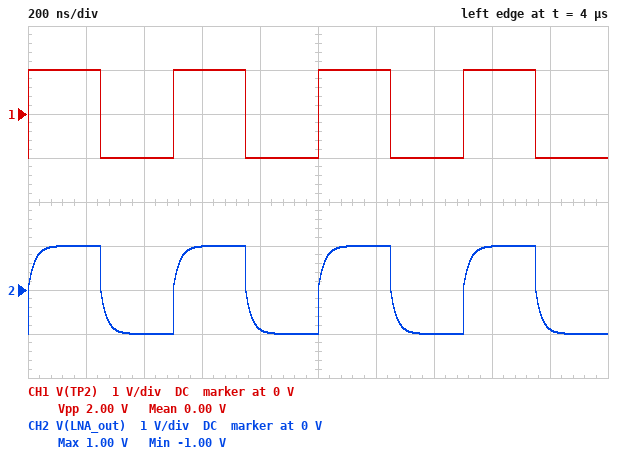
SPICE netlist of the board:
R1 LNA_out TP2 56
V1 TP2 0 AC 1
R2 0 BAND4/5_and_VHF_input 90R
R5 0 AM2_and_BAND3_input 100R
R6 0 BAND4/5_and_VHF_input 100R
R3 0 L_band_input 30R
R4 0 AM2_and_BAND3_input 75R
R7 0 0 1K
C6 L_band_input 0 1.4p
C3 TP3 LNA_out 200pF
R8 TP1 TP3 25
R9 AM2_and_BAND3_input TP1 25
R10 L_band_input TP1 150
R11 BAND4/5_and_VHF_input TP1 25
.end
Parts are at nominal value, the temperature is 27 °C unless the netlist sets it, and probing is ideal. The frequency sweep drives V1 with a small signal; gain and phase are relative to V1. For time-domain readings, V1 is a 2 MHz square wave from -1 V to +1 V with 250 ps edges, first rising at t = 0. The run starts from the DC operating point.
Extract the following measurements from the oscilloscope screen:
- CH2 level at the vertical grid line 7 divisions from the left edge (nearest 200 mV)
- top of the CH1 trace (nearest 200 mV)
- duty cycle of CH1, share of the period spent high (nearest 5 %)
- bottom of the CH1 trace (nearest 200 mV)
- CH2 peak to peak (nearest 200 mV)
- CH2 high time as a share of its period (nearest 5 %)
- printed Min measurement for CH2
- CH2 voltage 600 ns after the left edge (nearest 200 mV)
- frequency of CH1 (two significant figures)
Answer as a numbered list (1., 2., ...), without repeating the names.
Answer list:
1. -1.0 V
2. 1.0 V
3. 50 %
4. -1.0 V
5. 2.0 V
6. 50 %
7. -1.00 V
8. 1.0 V
9. 2.0 MHz
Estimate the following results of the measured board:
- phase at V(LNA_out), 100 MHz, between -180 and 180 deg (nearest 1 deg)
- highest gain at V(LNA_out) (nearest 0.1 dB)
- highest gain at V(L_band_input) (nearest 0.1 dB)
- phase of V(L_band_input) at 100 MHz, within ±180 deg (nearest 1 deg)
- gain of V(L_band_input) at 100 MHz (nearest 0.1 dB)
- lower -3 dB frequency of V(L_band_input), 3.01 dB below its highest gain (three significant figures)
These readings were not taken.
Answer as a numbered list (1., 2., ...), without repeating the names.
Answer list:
1. -4 deg
2. 0 dB
3. -27.1 dB
4. 3 deg
5. -27.1 dB
6. 7.19 MHz
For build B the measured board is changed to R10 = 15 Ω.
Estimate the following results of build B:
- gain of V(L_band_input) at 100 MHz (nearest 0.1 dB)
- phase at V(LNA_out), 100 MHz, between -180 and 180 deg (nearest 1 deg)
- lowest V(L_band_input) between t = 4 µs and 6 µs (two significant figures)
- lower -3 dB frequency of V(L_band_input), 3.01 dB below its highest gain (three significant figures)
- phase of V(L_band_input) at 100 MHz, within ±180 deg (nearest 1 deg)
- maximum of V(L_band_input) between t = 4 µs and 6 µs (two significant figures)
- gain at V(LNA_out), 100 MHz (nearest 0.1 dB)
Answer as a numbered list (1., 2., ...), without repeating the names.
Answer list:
1. -17.7 dB
2. -6 deg
3. -260 mV
4. 7.88 MHz
5. 4 deg
6. 260 mV
7. -6.9 dB
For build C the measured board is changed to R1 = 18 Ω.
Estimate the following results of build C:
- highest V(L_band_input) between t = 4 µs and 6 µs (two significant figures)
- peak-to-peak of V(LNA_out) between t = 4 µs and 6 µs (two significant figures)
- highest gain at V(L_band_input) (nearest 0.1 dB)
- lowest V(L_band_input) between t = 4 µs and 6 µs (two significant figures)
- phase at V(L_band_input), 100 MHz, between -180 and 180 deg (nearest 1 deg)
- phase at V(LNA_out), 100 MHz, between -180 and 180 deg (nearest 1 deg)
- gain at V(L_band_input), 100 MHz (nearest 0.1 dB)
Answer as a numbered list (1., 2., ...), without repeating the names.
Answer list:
1. 130 mV
2. 2.0 V
3. -23.4 dB
4. -130 mV
5. 5 deg
6. -2 deg
7. -23.5 dB
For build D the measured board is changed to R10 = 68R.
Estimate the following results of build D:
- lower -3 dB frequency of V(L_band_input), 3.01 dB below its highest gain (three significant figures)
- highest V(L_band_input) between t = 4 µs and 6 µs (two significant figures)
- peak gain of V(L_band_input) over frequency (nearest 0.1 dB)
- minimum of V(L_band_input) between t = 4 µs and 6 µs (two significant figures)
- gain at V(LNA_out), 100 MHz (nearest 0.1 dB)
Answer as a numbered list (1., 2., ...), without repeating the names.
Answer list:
1. 7.43 MHz
2. 150 mV
3. -22.6 dB
4. -150 mV
5. -6.4 dB
